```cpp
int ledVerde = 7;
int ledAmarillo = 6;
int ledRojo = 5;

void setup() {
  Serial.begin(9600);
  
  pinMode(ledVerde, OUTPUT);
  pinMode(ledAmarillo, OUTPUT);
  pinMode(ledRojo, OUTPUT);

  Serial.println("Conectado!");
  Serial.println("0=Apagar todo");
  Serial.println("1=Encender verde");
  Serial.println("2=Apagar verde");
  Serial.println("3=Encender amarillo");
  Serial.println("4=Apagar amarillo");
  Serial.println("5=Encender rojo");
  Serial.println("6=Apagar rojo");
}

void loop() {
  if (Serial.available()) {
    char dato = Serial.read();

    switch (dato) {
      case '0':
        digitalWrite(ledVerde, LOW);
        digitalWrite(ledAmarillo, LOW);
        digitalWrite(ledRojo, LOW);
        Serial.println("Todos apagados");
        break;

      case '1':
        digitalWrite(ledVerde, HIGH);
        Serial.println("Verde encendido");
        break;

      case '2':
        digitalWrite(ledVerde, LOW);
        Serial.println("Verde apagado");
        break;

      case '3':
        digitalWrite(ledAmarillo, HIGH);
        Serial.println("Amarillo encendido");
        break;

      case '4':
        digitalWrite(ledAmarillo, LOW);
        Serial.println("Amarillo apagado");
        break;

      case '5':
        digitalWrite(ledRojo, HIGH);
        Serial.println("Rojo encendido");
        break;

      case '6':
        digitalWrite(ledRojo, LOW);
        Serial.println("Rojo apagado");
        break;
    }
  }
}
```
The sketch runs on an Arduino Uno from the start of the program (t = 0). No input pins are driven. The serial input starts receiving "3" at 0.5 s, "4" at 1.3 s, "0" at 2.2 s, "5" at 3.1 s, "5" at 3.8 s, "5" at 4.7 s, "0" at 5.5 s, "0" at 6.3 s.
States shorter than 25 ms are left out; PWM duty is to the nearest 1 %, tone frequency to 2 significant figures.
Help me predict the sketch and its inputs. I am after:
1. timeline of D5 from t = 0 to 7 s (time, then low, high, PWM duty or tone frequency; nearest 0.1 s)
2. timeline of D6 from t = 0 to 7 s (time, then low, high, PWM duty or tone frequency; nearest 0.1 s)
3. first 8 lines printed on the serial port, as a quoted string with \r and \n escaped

0 s low; 3.1 s high; 5.5 s low
0 s low; 0.5 s high; 1.3 s low
"Conectado!\r\n0=Apagar todo\r\n1=Encender verde\r\n2=Apagar verde\r\n3=Encender amarillo\r\n4=Apagar amarillo\r\n5=Encender rojo\r\n6=Apagar rojo\r\n"
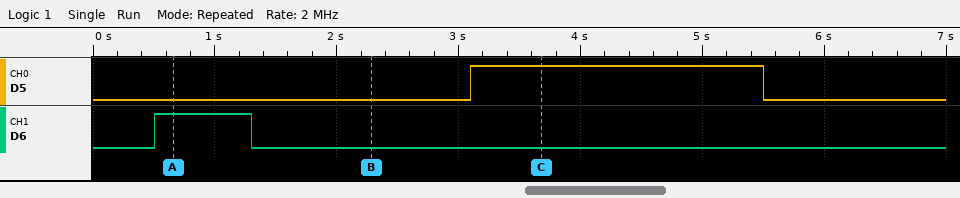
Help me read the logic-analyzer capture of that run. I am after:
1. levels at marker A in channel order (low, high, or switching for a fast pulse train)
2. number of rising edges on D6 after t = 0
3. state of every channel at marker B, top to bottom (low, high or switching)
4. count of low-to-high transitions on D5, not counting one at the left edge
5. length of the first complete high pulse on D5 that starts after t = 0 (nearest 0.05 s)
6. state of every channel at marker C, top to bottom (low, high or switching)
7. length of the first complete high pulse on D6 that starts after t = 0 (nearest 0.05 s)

D5 low, D6 high
1
D5 low, D6 low
1
2.40 s
D5 high, D6 low
0.80 s
